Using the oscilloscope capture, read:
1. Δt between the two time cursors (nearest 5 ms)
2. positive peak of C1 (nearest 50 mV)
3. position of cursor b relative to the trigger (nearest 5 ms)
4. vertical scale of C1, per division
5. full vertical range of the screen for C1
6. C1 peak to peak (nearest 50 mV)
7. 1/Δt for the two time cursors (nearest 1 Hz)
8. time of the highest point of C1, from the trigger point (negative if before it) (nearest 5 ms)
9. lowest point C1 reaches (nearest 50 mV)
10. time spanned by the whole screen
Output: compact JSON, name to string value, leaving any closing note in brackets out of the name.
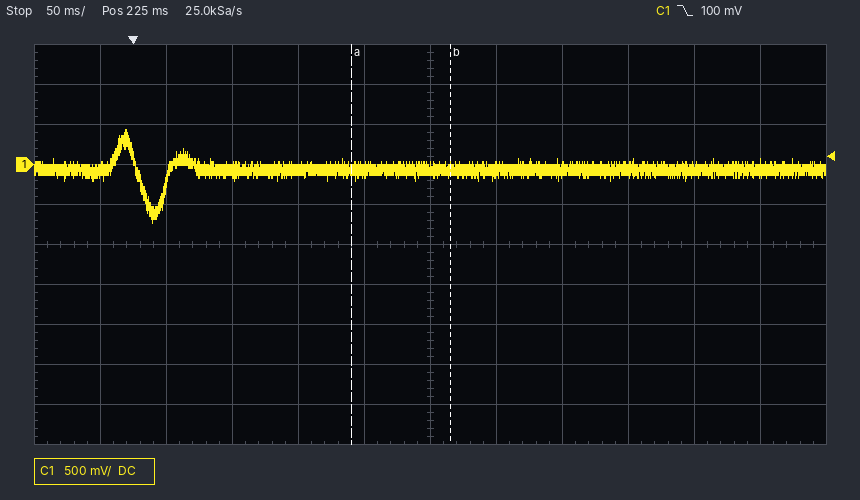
{"Δt between the two time cursors": "75 ms", "positive peak of C1": "450 mV", "position of cursor b relative to the trigger": "+240 ms", "vertical scale of C1, per division": "500 mV", "full vertical range of the screen for C1": "5 V", "C1 peak to peak": "1.15 V", "1/Δt for the two time cursors": "13 Hz", "time of the highest point of C1, from the trigger point (negative if before it)": "-5 ms", "lowest point C1 reaches": "-700 mV", "time spanned by the whole screen": "600 ms"}
